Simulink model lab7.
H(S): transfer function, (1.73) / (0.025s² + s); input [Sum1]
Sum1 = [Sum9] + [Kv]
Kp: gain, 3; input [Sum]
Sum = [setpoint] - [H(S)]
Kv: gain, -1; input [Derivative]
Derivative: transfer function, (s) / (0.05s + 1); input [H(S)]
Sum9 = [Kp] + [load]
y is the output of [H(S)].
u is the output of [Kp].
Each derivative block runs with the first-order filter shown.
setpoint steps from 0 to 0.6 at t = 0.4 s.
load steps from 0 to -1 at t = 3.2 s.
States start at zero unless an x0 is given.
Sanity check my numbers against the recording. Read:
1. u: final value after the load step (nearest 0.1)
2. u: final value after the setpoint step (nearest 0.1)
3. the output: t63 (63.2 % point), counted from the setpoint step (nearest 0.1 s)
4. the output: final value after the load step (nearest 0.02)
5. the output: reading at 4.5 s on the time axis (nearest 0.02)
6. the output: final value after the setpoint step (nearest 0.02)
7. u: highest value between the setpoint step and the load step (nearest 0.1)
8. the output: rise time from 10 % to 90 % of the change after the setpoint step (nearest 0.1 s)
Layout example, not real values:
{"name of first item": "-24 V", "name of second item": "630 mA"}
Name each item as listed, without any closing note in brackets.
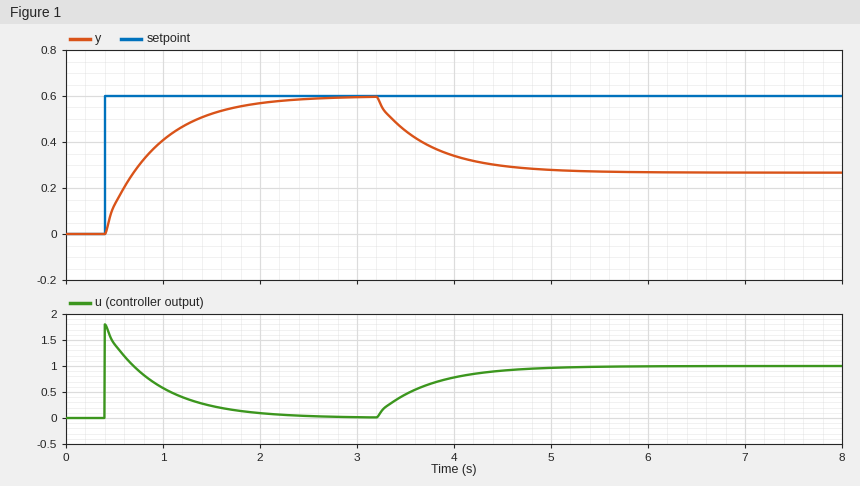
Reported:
{"u: final value after the load step": "1.0", "u: final value after the setpoint step": "0.0", "the output: t63 (63.2 % point), counted from the setpoint step": "0.5 s", "the output: final value after the load step": "0.26", "the output: reading at 4.5 s on the time axis": "0.30", "the output: final value after the setpoint step": "0.60", "u: highest value between the setpoint step and the load step": "1.8", "the output: rise time from 10 % to 90 % of the change after the setpoint step": "1.2 s"}
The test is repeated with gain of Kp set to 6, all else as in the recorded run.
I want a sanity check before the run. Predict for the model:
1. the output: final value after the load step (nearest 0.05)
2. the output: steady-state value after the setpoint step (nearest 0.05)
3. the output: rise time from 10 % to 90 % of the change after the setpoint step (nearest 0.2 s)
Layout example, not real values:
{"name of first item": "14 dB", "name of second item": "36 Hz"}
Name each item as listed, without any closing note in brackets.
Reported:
{"the output: final value after the load step": "0.45", "the output: steady-state value after the setpoint step": "0.60", "the output: rise time from 10 % to 90 % of the change after the setpoint step": "0.6 s"}
